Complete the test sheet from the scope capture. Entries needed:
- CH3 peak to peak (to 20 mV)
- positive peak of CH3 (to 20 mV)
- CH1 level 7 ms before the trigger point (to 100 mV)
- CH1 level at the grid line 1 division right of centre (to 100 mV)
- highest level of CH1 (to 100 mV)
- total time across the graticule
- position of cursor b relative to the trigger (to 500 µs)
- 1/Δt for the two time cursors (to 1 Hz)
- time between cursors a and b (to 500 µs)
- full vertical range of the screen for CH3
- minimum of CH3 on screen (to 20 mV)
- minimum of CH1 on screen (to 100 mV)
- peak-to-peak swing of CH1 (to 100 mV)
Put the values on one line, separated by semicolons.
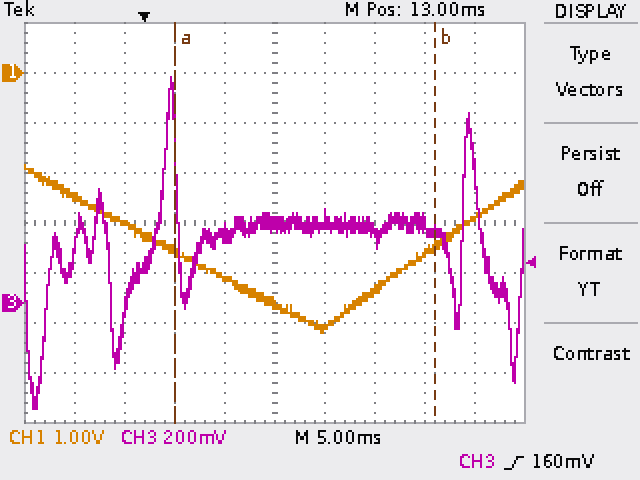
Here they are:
1.32 V; 900 mV; -2.5 V; -5.1 V; -1.8 V; 50 ms; +29.0 ms; 38 Hz; 26.0 ms; 1.6 V; -420 mV; -5.2 V; 3.4 V
